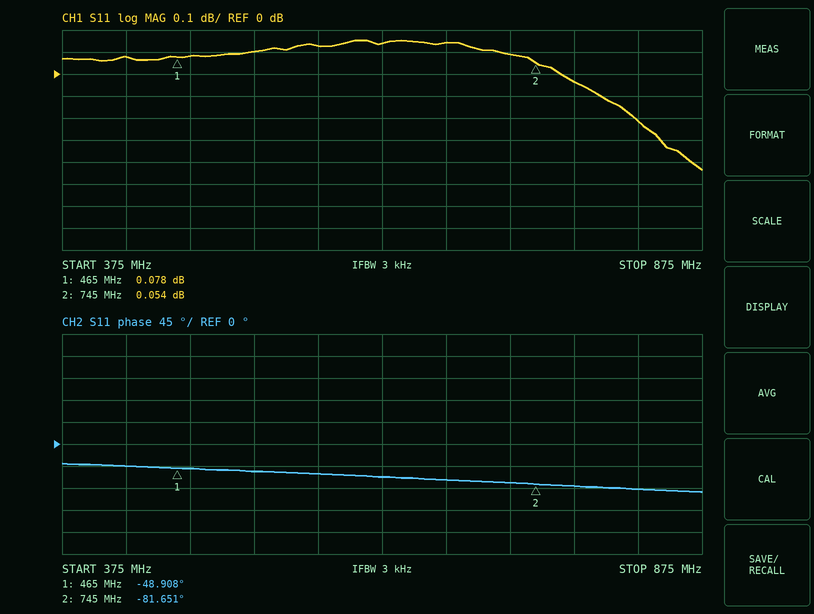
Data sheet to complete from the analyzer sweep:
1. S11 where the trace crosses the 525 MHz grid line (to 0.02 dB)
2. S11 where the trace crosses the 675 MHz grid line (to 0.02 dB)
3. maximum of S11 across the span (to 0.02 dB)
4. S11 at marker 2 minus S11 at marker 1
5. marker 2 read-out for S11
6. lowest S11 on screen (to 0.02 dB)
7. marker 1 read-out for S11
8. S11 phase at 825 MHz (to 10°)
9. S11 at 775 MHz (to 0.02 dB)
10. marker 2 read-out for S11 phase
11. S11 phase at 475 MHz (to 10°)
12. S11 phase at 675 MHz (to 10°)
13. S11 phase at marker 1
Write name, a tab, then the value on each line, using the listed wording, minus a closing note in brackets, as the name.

S11 where the trace crosses the 525 MHz grid line	0.10 dB
S11 where the trace crosses the 675 MHz grid line	0.14 dB
maximum of S11 across the span	0.16 dB
S11 at marker 2 minus S11 at marker 1	-0.024 dB
marker 2 read-out for S11	0.054 dB
lowest S11 on screen	-0.44 dB
marker 1 read-out for S11	0.078 dB
S11 phase at 825 MHz	-90°
S11 at 775 MHz	-0.04 dB
marker 2 read-out for S11 phase	-81.651°
S11 phase at 475 MHz	-50°
S11 phase at 675 MHz	-70°
S11 phase at marker 1	-48.908°
